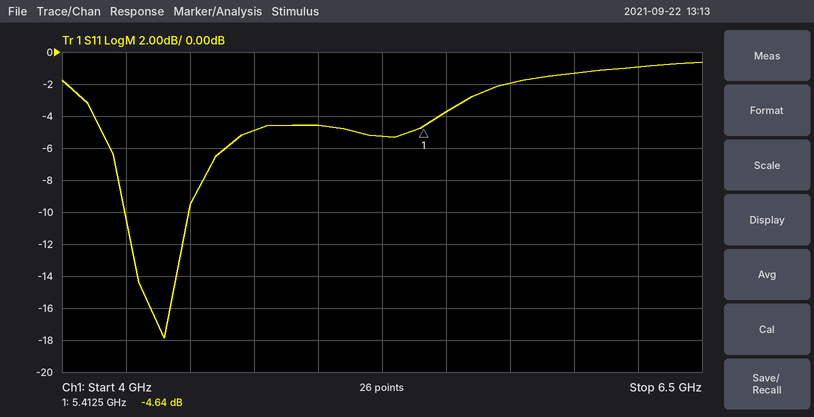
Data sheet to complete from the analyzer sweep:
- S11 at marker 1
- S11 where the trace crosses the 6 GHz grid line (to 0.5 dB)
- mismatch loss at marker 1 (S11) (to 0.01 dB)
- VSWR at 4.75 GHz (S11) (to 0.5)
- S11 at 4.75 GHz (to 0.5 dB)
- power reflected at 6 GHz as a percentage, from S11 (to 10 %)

-4.64 dB
-1.5 dB
1.83 dB
3.5
-5.0 dB
70 %
